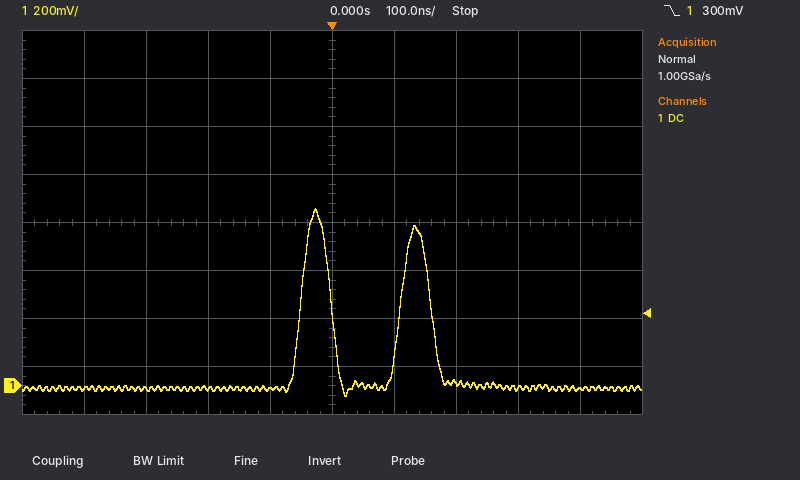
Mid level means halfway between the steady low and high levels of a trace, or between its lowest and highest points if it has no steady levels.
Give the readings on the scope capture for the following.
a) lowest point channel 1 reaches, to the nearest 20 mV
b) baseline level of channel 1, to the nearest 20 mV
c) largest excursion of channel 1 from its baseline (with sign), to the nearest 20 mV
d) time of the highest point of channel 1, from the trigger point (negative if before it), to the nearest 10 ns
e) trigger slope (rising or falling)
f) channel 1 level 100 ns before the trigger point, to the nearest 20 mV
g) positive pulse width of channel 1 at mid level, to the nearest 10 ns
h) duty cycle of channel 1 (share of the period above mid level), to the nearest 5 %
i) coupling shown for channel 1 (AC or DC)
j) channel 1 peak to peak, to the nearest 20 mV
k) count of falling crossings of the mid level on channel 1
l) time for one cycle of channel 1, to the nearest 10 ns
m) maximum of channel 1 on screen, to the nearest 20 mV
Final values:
-40 mV
0 mV
+740 mV
-30 ns
falling
-20 mV
50 ns
30 %
DC
780 mV
2
160 ns
740 mV
